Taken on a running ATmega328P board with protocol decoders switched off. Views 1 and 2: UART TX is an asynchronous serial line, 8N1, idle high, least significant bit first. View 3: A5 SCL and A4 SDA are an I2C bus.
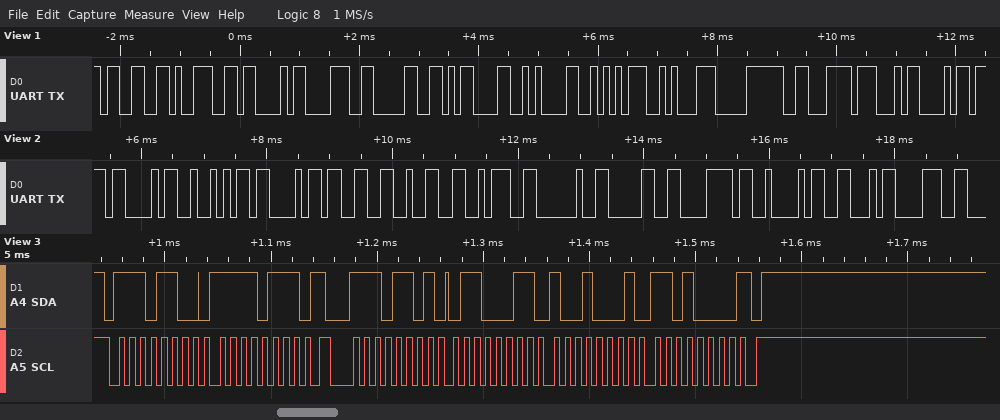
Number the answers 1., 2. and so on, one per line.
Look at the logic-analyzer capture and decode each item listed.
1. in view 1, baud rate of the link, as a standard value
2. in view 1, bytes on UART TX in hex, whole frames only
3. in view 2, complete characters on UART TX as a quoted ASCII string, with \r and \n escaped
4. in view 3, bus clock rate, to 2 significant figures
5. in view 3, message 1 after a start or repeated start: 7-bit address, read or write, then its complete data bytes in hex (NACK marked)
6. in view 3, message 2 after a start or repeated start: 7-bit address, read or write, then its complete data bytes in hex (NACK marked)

1. 9600 baud
2. 33 39 43 38 30 0D 0A AA 8A F0 C6 47 68
3. "CRC32: 0xBF8"
4. 100 kHz
5. 0x76 write: F7
6. 0x76 read: 63 91 D0 NACK
